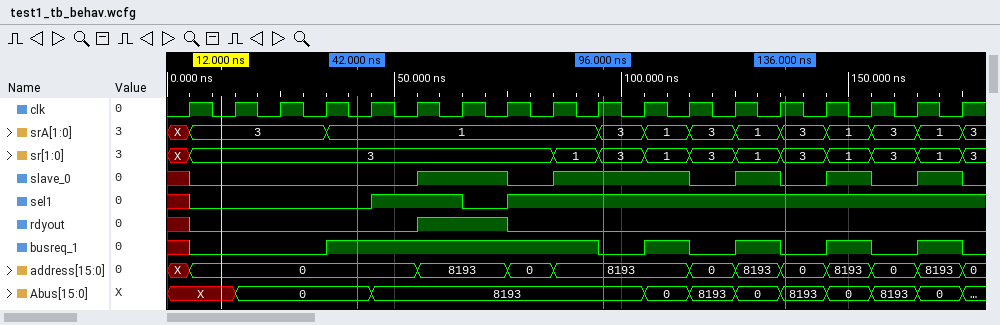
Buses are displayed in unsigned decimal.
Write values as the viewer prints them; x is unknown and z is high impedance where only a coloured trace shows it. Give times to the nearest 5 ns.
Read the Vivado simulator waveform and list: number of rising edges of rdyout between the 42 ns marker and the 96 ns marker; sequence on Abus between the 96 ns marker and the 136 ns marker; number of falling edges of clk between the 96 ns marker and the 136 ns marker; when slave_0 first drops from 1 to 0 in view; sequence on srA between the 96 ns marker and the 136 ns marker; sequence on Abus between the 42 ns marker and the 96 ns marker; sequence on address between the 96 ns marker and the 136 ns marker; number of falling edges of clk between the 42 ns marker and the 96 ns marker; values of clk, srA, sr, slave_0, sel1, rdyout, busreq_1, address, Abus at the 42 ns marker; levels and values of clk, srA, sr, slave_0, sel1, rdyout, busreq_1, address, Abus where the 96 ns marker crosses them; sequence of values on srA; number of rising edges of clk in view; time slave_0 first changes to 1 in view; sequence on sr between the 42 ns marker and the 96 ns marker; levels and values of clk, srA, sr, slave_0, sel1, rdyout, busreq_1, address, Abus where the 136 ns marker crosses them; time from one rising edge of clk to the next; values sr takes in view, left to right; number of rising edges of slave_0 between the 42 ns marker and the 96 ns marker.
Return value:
1
8193, 0, 8193, 0, 8193
4
75 ns
3, 1, 3, 1, 3
0, 8193
8193, 0, 8193, 0
5
clk=0, srA=1, sr=3, slave_0=0, sel1=0, rdyout=0, busreq_1=1, address=0, Abus=0
clk=1, srA=3, sr=3, slave_0=1, sel1=1, rdyout=0, busreq_1=0, address=8193, Abus=8193
X, 3, 1, 3, 1, 3, 1, 3, 1, 3, 1, 3
18
55 ns
3, 1, 3
clk=1, srA=3, sr=3, slave_0=0, sel1=1, rdyout=0, busreq_1=0, address=0, Abus=8193
10 ns
X, 3, 1, 3, 1, 3, 1, 3, 1, 3, 1, 3
2
